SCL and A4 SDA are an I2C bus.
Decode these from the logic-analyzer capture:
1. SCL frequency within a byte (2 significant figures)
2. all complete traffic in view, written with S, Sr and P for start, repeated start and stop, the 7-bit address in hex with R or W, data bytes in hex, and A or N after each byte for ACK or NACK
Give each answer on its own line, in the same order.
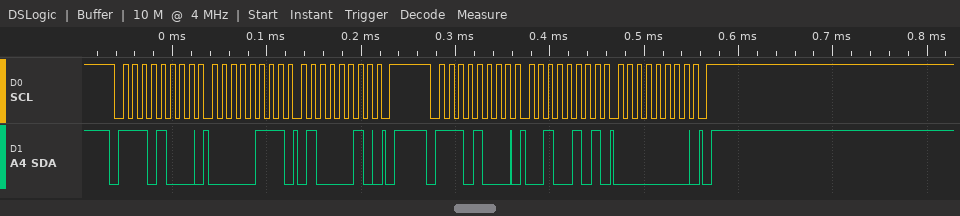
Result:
100 kHz
S 74W A 07 A 42 A P S 74W A 25 A 00 A P
